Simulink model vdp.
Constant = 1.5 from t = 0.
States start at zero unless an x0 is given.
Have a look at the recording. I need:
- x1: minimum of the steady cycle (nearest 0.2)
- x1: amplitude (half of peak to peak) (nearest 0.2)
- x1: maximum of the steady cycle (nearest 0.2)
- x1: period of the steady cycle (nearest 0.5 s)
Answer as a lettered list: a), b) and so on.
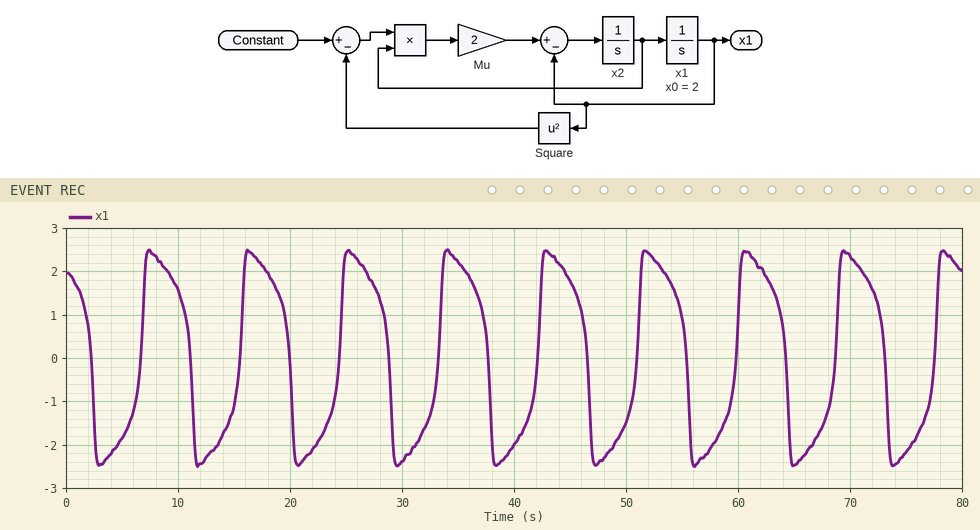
a) -2.4
b) 2.4
c) 2.4
d) 9.0 s
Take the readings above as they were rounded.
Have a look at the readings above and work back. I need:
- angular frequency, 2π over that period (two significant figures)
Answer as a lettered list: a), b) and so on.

a) 0.70 rad/s
